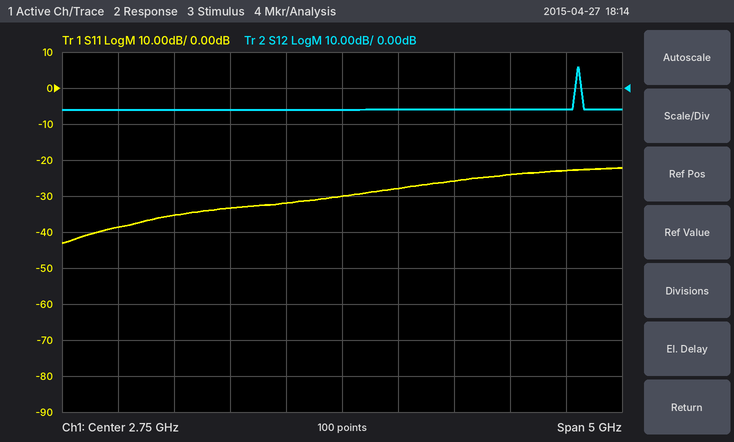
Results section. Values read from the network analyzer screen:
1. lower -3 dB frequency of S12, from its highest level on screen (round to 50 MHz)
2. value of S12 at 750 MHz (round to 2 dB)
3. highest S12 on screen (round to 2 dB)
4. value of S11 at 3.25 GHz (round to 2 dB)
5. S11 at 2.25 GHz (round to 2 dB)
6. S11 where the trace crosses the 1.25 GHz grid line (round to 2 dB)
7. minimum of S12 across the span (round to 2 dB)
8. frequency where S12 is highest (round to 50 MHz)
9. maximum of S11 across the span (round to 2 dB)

4.85 GHz
-6 dB
6 dB
-28 dB
-32 dB
-36 dB
-6 dB
4.85 GHz
-22 dB
